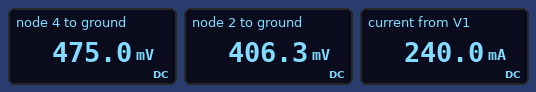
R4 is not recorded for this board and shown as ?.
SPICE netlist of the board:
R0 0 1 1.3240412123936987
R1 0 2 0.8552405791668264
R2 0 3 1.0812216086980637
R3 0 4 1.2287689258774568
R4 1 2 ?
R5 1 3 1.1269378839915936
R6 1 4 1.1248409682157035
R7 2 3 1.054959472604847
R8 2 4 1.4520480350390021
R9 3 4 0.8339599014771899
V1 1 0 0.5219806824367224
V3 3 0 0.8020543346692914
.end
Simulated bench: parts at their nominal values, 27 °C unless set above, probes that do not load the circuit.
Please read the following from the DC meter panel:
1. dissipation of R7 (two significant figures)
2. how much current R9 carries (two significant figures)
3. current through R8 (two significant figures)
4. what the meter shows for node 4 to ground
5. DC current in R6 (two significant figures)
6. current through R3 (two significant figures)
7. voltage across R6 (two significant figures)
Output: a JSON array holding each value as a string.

["150 mW", "390 mA", "47 mA", "475.0 mV", "42 mA", "390 mA", "47 mV"]
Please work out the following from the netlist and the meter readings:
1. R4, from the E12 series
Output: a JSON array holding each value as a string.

["2.2 Ω"]
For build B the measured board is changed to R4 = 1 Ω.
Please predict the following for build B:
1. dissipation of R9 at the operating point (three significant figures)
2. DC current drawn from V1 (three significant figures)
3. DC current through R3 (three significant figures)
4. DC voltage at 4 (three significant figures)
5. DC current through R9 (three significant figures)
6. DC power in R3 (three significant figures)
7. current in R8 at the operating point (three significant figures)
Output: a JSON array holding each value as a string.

["126 mW", "283 mA", "389 mA", "478 mV", "388 mA", "186 mW", "37.8 mA"]
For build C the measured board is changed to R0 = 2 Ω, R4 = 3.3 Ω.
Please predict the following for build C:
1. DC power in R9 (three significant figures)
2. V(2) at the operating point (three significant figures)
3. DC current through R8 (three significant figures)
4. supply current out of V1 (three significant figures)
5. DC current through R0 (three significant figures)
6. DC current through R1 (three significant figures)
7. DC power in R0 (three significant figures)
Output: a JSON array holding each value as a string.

["129 mW", "400 mV", "50.6 mA", "92.1 mA", "261 mA", "468 mA", "136 mW"]
